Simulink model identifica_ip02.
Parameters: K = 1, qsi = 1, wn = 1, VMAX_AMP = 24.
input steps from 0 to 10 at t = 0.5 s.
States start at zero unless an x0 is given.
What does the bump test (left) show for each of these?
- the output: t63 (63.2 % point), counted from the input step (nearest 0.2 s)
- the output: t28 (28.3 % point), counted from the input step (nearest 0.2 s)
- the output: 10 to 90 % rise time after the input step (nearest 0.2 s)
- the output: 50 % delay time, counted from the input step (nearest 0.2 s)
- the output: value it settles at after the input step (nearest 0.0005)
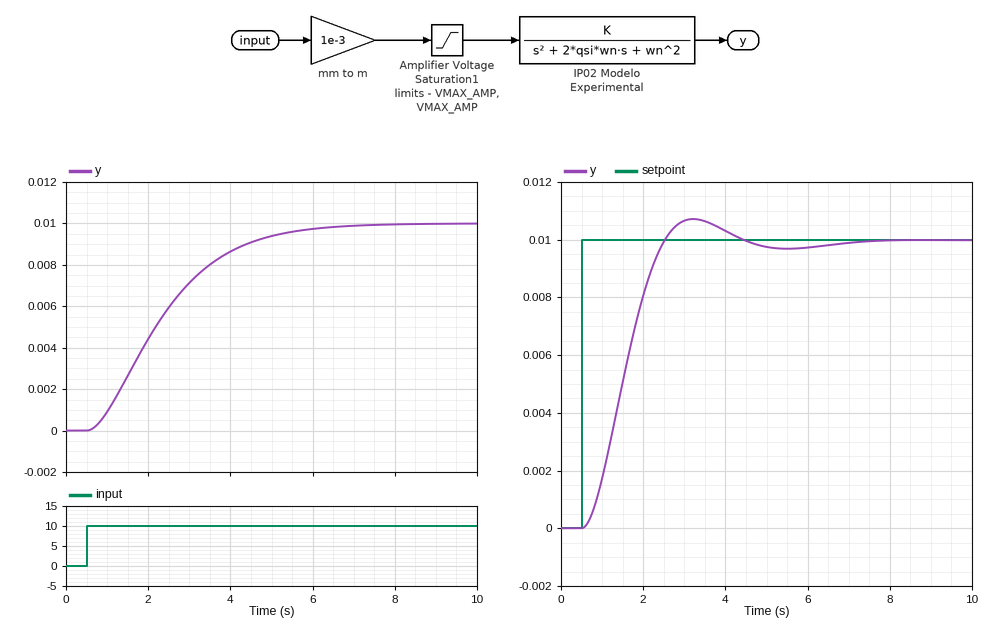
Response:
2.2 s
1.0 s
3.4 s
1.6 s
0.0100
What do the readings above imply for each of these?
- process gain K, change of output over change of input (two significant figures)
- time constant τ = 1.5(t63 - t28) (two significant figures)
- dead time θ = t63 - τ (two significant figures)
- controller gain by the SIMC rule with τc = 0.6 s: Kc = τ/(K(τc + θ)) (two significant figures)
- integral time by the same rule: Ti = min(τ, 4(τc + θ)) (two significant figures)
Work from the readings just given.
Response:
0.0010
1.8 s
0.40 s
1800
1.8 s
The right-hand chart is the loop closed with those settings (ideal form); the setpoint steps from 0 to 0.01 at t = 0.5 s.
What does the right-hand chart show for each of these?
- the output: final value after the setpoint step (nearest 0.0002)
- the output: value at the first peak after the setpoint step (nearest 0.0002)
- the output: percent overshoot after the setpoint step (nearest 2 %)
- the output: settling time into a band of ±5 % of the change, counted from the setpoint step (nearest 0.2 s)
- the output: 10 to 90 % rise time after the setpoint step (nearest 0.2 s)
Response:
0.0100
0.0108
8 %
3.2 s
1.4 s
